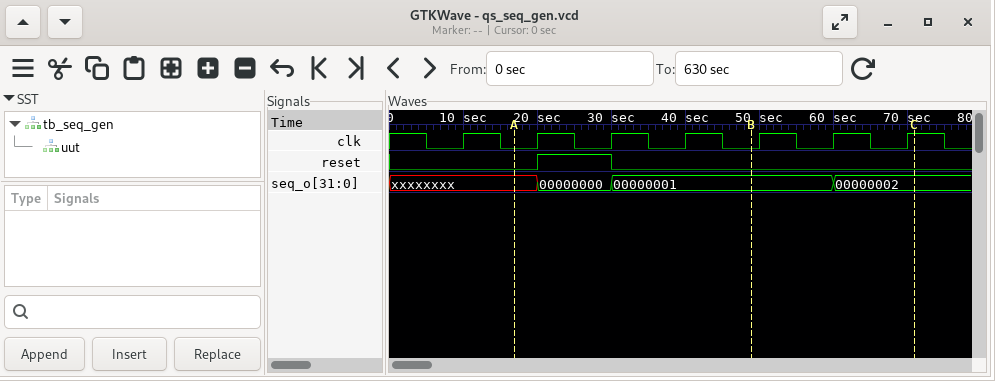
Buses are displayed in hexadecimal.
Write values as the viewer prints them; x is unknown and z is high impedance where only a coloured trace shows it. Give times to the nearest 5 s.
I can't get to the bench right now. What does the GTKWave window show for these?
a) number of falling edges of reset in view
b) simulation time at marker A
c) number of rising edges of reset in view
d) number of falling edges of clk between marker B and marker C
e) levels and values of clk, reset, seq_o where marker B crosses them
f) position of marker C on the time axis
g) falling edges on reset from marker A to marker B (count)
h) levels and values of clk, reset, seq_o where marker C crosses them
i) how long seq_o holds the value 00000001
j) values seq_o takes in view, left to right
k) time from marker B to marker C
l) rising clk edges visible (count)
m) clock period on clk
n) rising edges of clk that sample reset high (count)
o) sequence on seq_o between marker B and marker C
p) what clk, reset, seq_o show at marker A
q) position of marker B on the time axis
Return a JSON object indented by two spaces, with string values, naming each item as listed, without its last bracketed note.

{
  "number of falling edges of reset in view": "1",
  "simulation time at marker A": "15 s",
  "number of rising edges of reset in view": "1",
  "number of falling edges of clk between marker B and marker C": "2",
  "levels and values of clk, reset, seq_o where marker B crosses them": "clk=0, reset=0, seq_o=00000001",
  "position of marker C on the time axis": "70 s",
  "falling edges on reset from marker A to marker B": "1",
  "levels and values of clk, reset, seq_o where marker C crosses them": "clk=1, reset=0, seq_o=00000002",
  "how long seq_o holds the value 00000001": "30 s",
  "values seq_o takes in view, left to right": "xxxxxxxx, 00000000, 00000001, 00000002",
  "time from marker B to marker C": "20 s",
  "rising clk edges visible": "7",
  "clock period on clk": "10 s",
  "rising edges of clk that sample reset high": "1",
  "sequence on seq_o between marker B and marker C": "00000001, 00000002",
  "what clk, reset, seq_o show at marker A": "clk=0, reset=0, seq_o=xxxxxxxx",
  "position of marker B on the time axis": "50 s"
}
